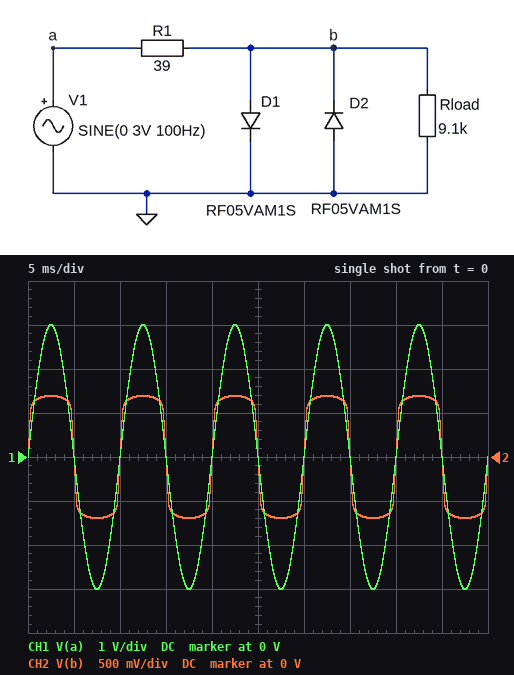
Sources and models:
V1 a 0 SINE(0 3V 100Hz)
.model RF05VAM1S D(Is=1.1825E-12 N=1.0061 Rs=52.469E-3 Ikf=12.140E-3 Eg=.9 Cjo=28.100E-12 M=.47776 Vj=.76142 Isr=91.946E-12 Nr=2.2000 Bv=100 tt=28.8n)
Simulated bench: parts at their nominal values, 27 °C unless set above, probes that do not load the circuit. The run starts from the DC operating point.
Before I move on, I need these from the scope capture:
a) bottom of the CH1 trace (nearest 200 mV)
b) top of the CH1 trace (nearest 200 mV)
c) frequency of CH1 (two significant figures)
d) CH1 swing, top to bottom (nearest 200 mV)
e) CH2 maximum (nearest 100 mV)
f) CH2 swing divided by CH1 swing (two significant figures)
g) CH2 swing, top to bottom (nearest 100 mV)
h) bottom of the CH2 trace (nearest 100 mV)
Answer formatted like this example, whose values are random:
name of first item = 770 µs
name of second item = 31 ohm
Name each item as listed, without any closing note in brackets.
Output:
bottom of the CH1 trace = -3.0 V
top of the CH1 trace = 3.0 V
frequency of CH1 = 100 Hz
CH1 swing, top to bottom = 6.0 V
CH2 maximum = 700 mV
CH2 swing divided by CH1 swing = 0.23
CH2 swing, top to bottom = 1.4 V
bottom of the CH2 trace = -700 mV
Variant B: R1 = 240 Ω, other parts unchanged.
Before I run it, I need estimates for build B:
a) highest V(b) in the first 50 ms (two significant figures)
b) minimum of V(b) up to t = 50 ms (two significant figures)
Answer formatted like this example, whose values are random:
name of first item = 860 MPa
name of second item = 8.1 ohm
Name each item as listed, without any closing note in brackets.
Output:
highest V(b) in the first 50 ms = 620 mV
minimum of V(b) up to t = 50 ms = -620 mV
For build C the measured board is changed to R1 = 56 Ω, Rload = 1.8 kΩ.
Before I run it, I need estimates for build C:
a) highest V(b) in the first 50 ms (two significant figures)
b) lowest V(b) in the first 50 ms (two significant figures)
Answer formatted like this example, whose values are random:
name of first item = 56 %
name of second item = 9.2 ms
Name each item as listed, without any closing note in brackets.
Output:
highest V(b) in the first 50 ms = 680 mV
lowest V(b) in the first 50 ms = -680 mV
